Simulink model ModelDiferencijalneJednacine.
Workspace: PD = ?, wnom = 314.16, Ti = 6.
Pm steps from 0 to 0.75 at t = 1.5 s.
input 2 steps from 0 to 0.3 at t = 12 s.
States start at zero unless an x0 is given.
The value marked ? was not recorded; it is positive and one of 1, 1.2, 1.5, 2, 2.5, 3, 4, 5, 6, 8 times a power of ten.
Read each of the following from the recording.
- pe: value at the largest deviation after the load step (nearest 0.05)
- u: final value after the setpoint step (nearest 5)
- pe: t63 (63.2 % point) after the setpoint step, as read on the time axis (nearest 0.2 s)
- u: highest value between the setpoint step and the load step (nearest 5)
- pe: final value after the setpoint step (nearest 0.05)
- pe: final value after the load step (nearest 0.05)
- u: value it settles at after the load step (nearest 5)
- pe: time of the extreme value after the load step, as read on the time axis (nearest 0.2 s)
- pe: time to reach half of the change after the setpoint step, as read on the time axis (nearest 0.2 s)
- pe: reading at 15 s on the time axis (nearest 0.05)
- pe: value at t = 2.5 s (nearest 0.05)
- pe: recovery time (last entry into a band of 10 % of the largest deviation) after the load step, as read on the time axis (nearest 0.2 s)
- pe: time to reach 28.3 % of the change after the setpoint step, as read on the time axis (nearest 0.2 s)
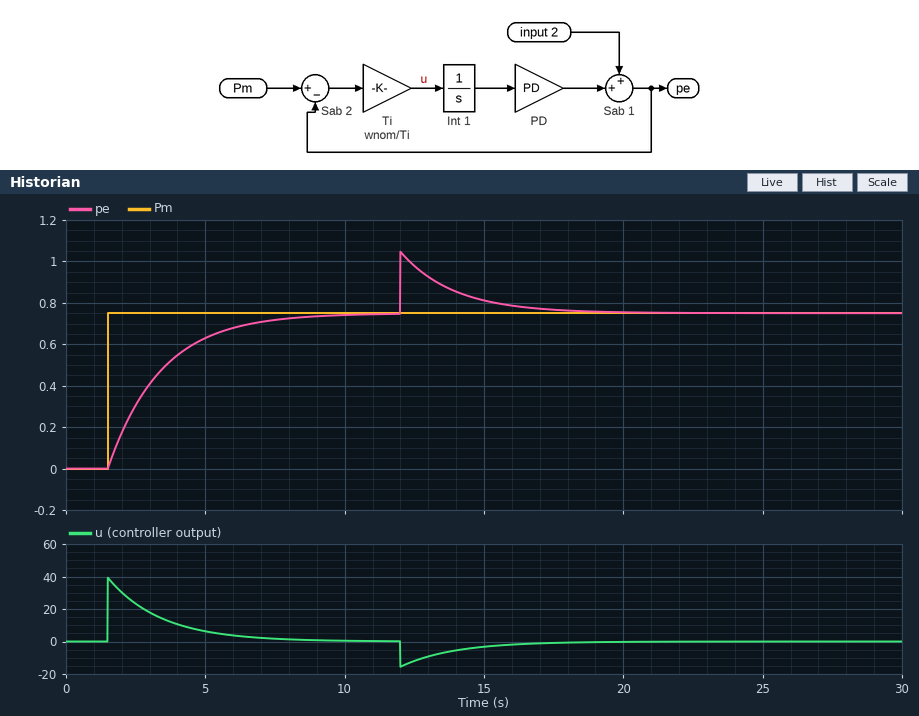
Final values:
1.05
0
3.4 s
40
0.75
0.75
0
12.0 s
2.8 s
0.80
0.30
16.4 s
2.2 s
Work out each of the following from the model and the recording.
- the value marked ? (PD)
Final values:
0.01
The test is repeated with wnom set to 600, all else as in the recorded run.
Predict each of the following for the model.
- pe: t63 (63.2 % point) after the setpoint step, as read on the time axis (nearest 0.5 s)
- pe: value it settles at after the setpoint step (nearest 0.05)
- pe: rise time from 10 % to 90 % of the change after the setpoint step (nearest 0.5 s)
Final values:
2.5 s
0.75
2.0 s
